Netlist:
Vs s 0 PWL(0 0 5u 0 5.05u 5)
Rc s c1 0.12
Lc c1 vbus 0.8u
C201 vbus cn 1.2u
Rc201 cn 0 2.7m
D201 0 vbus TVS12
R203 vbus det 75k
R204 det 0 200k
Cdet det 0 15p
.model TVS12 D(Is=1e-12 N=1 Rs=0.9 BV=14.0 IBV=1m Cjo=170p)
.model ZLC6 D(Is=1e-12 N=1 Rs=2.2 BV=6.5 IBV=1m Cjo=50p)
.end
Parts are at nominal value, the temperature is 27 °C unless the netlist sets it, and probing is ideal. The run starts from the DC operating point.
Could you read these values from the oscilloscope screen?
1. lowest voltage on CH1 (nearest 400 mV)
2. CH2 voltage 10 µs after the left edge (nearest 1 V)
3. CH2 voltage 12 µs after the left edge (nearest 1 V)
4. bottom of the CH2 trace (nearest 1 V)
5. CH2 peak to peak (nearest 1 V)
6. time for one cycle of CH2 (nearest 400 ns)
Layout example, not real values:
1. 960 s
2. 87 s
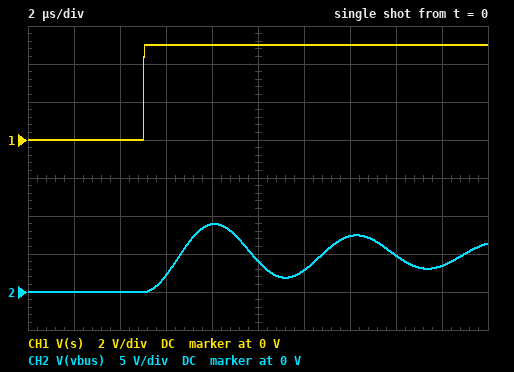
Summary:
1. 0 V
2. 4 V
3. 3 V
4. 0 V
5. 9 V
6. 6.0 µs
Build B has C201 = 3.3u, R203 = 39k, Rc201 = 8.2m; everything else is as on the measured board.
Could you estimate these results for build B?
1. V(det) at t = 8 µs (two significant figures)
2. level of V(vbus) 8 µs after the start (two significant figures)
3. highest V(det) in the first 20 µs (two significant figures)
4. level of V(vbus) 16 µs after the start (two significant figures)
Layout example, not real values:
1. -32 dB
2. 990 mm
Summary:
1. 3.6 V
2. 5.5 V
3. 6.8 V
4. 3.0 V
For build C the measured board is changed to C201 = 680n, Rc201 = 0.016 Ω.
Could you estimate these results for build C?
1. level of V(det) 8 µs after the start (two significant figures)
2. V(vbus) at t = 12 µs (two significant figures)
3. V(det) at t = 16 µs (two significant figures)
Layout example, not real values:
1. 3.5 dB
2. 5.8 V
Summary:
1. 5.5 V
2. 7.8 V
3. 3.4 V
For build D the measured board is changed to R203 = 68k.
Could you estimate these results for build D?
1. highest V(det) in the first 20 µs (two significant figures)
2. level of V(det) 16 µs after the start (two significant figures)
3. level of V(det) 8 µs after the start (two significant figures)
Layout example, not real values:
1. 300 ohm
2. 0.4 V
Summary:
1. 6.0 V
2. 4.5 V
3. 5.3 V
